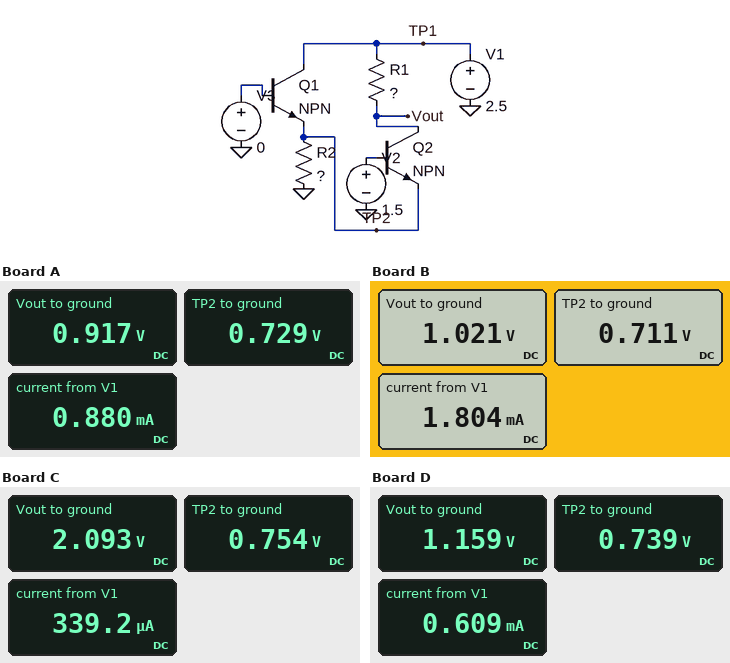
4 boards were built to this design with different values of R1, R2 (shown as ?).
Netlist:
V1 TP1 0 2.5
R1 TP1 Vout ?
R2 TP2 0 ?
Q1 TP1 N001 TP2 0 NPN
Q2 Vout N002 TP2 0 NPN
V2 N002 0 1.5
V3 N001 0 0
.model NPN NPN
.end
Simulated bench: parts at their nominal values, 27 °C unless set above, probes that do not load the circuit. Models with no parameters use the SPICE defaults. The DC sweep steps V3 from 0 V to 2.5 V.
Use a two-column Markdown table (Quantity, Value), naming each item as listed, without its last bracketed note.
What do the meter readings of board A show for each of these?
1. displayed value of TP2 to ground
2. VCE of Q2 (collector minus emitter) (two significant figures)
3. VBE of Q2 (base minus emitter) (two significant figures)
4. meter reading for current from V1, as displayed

| Quantity | Value |
|---|---|
| displayed value of TP2 to ground | 0.729 V |
| VCE of Q2 (collector minus emitter) | 190 mV |
| VBE of Q2 (base minus emitter) | 770 mV |
| meter reading for current from V1, as displayed | 0.880 mA |
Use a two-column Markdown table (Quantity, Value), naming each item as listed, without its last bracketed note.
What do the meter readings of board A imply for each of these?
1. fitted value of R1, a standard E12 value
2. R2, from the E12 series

| Quantity | Value |
|---|---|
| fitted value of R1, a standard E12 value | 1.8 kΩ |
| R2, from the E12 series | 820 Ω |
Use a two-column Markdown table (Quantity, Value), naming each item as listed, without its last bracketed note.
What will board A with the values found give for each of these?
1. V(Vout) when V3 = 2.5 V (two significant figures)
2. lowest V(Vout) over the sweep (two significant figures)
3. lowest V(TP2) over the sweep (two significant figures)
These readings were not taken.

| Quantity | Value |
|---|---|
| V(Vout) when V3 = 2.5 V | 2.5 V |
| lowest V(Vout) over the sweep | 920 mV |
| lowest V(TP2) over the sweep | 730 mV |
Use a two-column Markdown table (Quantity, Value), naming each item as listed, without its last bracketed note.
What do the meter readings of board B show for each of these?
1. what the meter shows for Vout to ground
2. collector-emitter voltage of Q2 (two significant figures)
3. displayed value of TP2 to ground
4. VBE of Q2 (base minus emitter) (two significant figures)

| Quantity | Value |
|---|---|
| what the meter shows for Vout to ground | 1.021 V |
| collector-emitter voltage of Q2 | 310 mV |
| displayed value of TP2 to ground | 0.711 V |
| VBE of Q2 (base minus emitter) | 790 mV |
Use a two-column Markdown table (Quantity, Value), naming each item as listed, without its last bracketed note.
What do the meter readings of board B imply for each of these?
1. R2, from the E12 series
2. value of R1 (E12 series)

| Quantity | Value |
|---|---|
| R2, from the E12 series | 390 Ω |
| value of R1 | 820 Ω |
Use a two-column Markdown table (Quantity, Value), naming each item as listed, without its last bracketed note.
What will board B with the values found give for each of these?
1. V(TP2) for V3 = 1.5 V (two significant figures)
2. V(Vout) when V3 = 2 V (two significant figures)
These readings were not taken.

| Quantity | Value |
|---|---|
| V(TP2) for V3 = 1.5 V | 730 mV |
| V(Vout) when V3 = 2 V | 2.5 V |
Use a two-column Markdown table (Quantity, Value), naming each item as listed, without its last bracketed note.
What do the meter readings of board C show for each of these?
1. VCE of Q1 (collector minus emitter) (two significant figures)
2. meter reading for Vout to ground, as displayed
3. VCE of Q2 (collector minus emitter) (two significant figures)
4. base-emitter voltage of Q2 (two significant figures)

| Quantity | Value |
|---|---|
| VCE of Q1 (collector minus emitter) | 1.7 V |
| meter reading for Vout to ground, as displayed | 2.093 V |
| VCE of Q2 (collector minus emitter) | 1.3 V |
| base-emitter voltage of Q2 | 750 mV |
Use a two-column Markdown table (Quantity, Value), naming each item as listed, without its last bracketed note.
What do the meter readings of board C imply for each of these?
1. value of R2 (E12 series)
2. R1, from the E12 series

| Quantity | Value |
|---|---|
| value of R2 | 2.2 kΩ |
| R1, from the E12 series | 1.2 kΩ |
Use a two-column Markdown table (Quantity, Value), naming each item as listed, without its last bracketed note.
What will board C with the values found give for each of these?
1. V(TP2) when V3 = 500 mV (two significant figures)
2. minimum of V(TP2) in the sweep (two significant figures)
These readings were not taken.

| Quantity | Value |
|---|---|
| V(TP2) when V3 = 500 mV | 750 mV |
| minimum of V(TP2) in the sweep | 750 mV |
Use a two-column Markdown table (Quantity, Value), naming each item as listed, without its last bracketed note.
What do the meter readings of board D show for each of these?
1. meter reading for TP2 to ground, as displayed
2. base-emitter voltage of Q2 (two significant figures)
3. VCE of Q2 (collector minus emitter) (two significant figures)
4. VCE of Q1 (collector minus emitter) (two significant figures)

| Quantity | Value |
|---|---|
| meter reading for TP2 to ground, as displayed | 0.739 V |
| base-emitter voltage of Q2 | 760 mV |
| VCE of Q2 (collector minus emitter) | 420 mV |
| VCE of Q1 (collector minus emitter) | 1.8 V |
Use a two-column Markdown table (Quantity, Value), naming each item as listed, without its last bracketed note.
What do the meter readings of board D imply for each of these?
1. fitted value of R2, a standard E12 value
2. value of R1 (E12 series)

| Quantity | Value |
|---|---|
| fitted value of R2, a standard E12 value | 1.2 kΩ |
| value of R1 | 2.2 kΩ |
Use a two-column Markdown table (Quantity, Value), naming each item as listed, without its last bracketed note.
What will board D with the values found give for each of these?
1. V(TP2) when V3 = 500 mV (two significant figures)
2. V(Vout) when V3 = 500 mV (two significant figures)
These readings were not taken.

| Quantity | Value |
|---|---|
| V(TP2) when V3 = 500 mV | 740 mV |
| V(Vout) when V3 = 500 mV | 1.2 V |
